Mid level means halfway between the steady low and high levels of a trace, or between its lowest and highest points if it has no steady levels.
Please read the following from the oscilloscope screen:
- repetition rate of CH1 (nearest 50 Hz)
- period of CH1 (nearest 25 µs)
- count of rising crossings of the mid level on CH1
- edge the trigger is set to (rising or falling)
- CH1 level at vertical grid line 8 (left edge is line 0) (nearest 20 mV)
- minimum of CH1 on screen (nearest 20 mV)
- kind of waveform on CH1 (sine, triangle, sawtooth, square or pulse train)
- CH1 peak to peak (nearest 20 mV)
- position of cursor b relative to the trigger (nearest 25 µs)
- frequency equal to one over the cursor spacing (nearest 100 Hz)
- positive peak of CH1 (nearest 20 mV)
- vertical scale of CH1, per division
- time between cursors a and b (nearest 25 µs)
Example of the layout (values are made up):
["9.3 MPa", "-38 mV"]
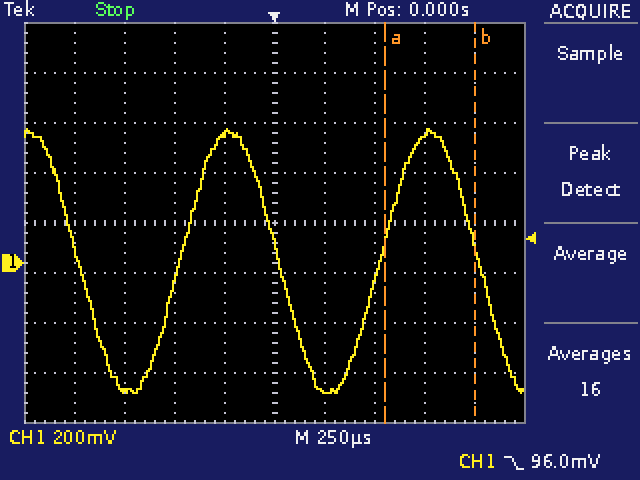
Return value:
["1.00 kHz", "1.000 ms", "2", "falling", "520 mV", "-520 mV", "sine", "1.06 V", "+1.000 ms", "2.2 kHz", "540 mV", "200 mV", "450 µs"]
